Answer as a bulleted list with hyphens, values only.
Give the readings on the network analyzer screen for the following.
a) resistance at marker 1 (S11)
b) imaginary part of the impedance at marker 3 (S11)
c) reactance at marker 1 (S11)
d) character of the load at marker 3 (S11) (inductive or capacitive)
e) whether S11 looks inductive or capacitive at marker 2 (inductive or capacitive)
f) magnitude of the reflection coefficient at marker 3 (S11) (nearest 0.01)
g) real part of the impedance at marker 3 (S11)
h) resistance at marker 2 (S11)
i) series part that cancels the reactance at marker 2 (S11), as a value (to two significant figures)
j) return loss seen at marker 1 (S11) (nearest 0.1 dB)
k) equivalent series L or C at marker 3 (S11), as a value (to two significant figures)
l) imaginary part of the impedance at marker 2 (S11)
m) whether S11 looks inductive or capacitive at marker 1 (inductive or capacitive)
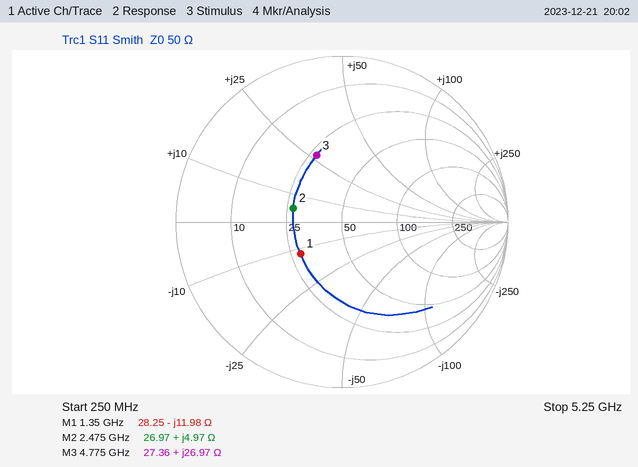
- 28.25 Ω
- +26.97 Ω
- -11.98 Ω
- inductive
- inductive
- 0.43
- 27.36 Ω
- 26.97 Ω
- 13 pF
- 10.1 dB
- 900 pH
- +4.97 Ω
- capacitive
